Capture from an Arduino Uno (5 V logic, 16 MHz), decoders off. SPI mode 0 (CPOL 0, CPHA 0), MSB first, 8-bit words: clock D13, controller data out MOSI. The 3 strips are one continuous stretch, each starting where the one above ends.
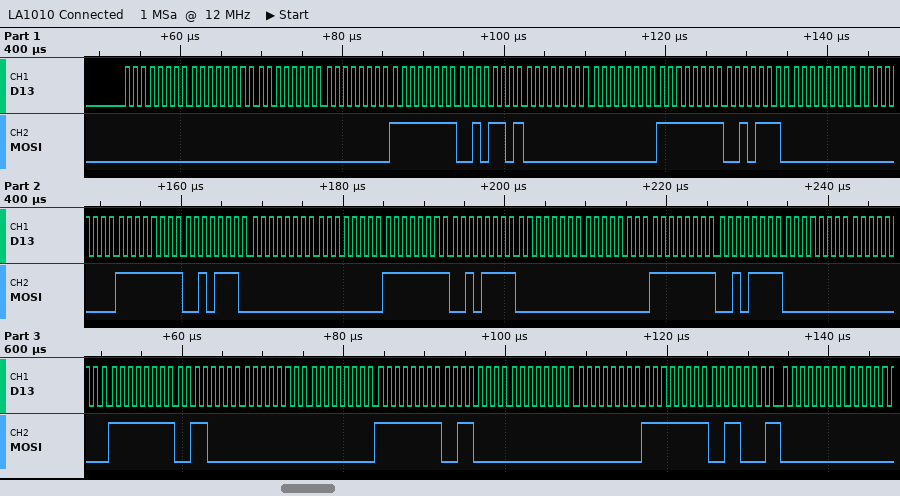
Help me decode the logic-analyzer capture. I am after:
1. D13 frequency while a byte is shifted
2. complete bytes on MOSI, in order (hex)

1 MHz
00 00 00 00 FF 2D 00 00 FF 2E 00 00 FF 2E 00 00 FF 2F 00 00 FF 2F 00 00 FF 30 00 00 FF 30 00 00 FF 31 00
